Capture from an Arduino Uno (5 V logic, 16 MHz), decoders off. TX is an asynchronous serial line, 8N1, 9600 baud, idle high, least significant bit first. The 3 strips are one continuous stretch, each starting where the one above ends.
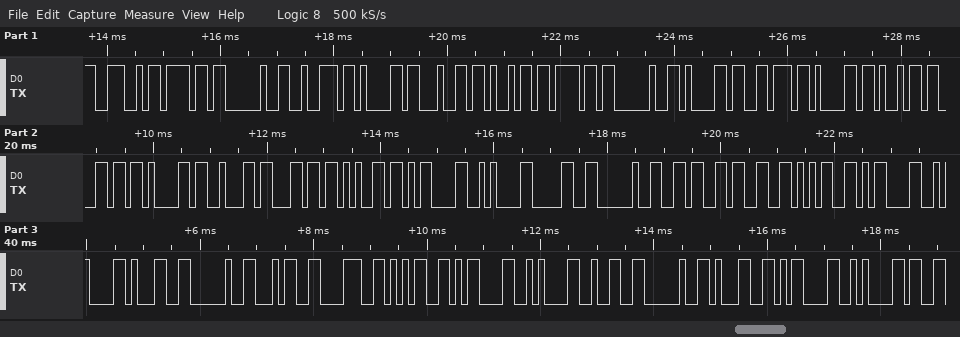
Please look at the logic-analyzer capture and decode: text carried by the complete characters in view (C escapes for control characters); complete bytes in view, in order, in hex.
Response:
"No radio available\r\n0 635\r\n1 485\r\n2 1\r\n"
4E 6F 20 72 61 64 69 6F 20 61 76 61 69 6C 61 62 6C 65 0D 0A 30 20 36 33 35 0D 0A 31 20 34 38 35 0D 0A 32 20 31 0D 0A
